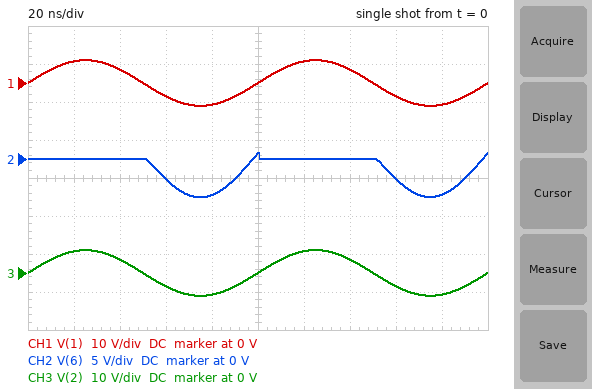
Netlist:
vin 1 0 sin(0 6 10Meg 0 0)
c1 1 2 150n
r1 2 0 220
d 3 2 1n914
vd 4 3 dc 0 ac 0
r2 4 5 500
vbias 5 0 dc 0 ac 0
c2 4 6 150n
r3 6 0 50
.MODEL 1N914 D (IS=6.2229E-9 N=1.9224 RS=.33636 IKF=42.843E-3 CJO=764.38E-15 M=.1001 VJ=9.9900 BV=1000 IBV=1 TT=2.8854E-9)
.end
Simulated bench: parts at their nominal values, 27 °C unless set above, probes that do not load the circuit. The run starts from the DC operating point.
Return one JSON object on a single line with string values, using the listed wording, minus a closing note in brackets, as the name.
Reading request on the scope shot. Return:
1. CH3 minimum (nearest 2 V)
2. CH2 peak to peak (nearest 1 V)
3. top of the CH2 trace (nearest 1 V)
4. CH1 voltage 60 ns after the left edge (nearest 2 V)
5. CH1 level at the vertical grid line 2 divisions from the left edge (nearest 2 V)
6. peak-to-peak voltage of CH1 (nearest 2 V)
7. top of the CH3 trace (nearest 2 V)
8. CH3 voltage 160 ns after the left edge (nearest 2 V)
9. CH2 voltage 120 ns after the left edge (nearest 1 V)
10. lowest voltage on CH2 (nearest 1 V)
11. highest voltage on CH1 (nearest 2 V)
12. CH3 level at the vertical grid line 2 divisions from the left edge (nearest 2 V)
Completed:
{"CH3 minimum": "-6 V", "CH2 peak to peak": "6 V", "top of the CH2 trace": "1 V", "CH1 voltage 60 ns after the left edge": "-4 V", "CH1 level at the vertical grid line 2 divisions from the left edge": "4 V", "peak-to-peak voltage of CH1": "12 V", "top of the CH3 trace": "6 V", "CH3 voltage 160 ns after the left edge": "-4 V", "CH2 voltage 120 ns after the left edge": "0 V", "lowest voltage on CH2": "-5 V", "highest voltage on CH1": "6 V", "CH3 level at the vertical grid line 2 divisions from the left edge": "4 V"}
